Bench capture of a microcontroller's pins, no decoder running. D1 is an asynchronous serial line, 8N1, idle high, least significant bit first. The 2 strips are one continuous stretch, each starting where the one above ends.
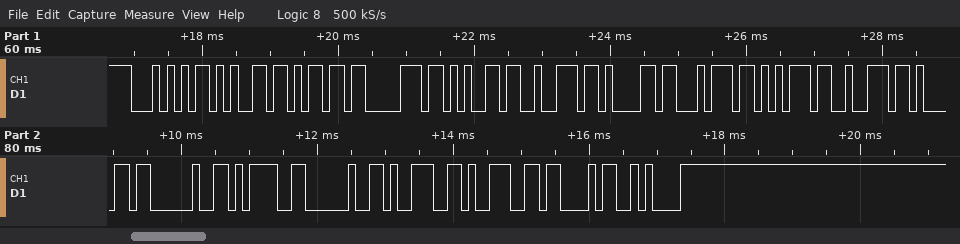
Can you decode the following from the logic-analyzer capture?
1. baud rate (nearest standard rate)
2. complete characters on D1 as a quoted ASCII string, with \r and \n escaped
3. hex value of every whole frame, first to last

9600 baud
"Temperatura = 99C\n"
0x54 0x65 0x6D 0x70 0x65 0x72 0x61 0x74 0x75 0x72 0x61 0x20 0x3D 0x20 0x39 0x39 0x43 0x0A
